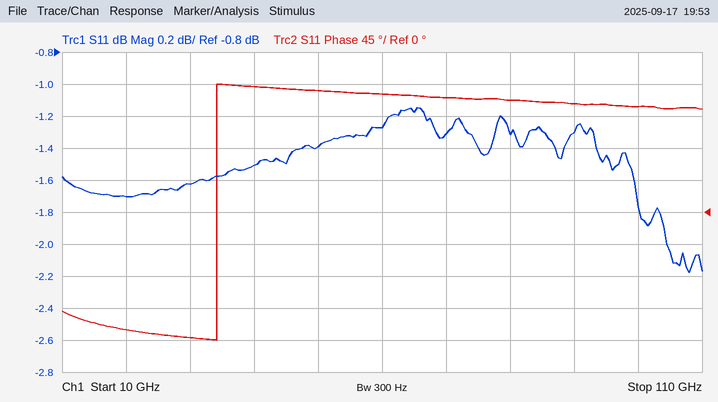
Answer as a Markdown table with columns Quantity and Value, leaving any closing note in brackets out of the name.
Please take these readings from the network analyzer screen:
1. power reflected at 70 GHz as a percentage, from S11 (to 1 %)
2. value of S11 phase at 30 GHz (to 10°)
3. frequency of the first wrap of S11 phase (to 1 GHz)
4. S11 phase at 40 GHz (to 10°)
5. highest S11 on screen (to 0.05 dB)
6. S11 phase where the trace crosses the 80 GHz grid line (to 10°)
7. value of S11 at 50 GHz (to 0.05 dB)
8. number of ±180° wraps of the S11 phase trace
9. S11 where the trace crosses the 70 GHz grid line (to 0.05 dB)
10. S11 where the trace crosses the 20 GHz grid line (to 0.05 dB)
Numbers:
| Quantity | Value |
|---|---|
| power reflected at 70 GHz as a percentage, from S11 | 74 % |
| value of S11 phase at 30 GHz | -180° |
| frequency of the first wrap of S11 phase | 34 GHz |
| S11 phase at 40 GHz | 180° |
| highest S11 on screen | -1.15 dB |
| S11 phase where the trace crosses the 80 GHz grid line | 160° |
| value of S11 at 50 GHz | -1.40 dB |
| number of ±180° wraps of the S11 phase trace | 1 |
| S11 where the trace crosses the 70 GHz grid line | -1.30 dB |
| S11 where the trace crosses the 20 GHz grid line | -1.70 dB |
